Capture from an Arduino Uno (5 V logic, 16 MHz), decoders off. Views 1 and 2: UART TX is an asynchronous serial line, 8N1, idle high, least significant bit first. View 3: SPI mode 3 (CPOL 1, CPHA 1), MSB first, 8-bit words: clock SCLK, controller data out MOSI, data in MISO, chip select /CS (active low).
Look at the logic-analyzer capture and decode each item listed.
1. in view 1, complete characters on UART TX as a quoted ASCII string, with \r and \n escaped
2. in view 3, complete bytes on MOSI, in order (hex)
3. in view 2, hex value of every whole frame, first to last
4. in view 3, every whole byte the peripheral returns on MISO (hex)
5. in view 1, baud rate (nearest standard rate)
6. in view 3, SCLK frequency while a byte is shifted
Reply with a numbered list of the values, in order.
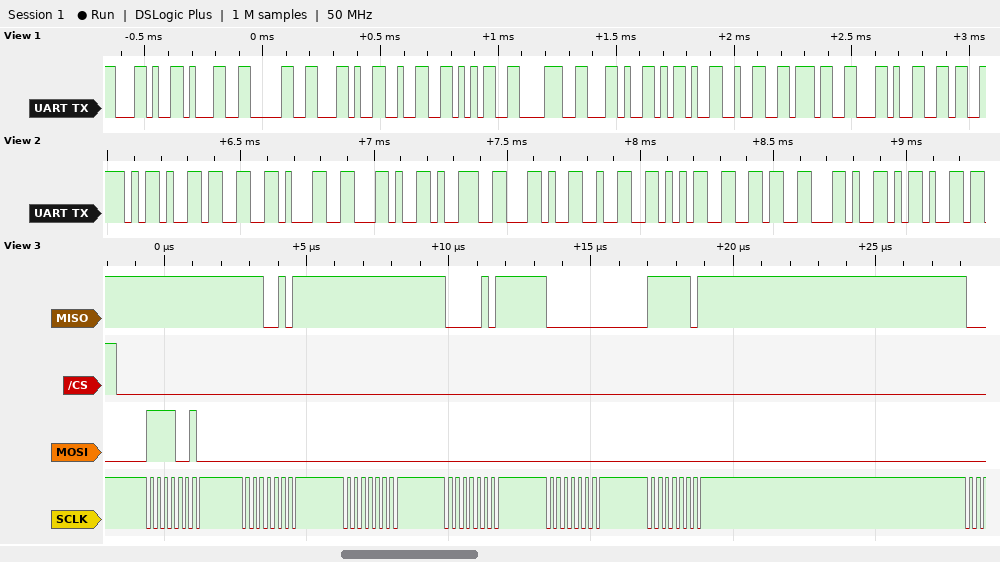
1. ",10,258,-27,6"
2. 0xF2 0x00 0x00 0x00 0x00 0x00
3. 0x2D 0x33 0x31 0x2C 0x39 0x2C 0x32 0x35 0x36 0x2C 0x2D
4. 0xFF 0xE5 0xFF 0x05 0x00 0xFD
5. 38400 baud
6. 4 MHz
